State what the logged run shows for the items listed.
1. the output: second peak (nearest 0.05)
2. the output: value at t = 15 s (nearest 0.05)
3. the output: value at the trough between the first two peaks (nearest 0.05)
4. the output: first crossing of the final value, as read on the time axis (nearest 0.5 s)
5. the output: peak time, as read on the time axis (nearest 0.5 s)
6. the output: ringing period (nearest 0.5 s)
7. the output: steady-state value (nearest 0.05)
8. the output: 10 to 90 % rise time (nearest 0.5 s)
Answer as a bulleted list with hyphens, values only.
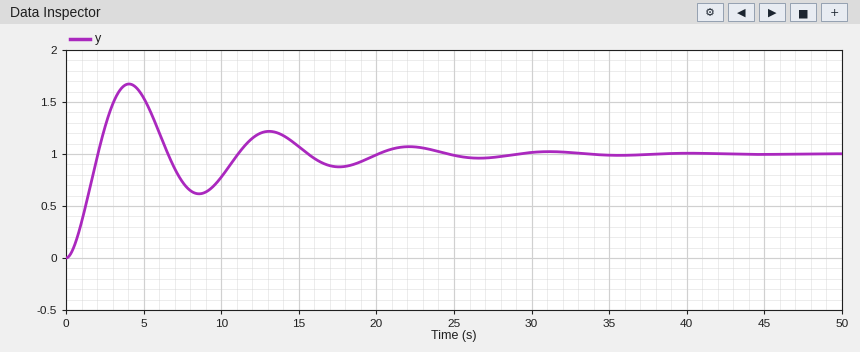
- 1.20
- 1.05
- 0.60
- 2.0 s
- 4.0 s
- 9.0 s
- 1.00
- 1.5 s
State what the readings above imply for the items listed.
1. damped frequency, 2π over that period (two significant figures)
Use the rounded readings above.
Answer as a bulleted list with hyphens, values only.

- 0.70 rad/s
